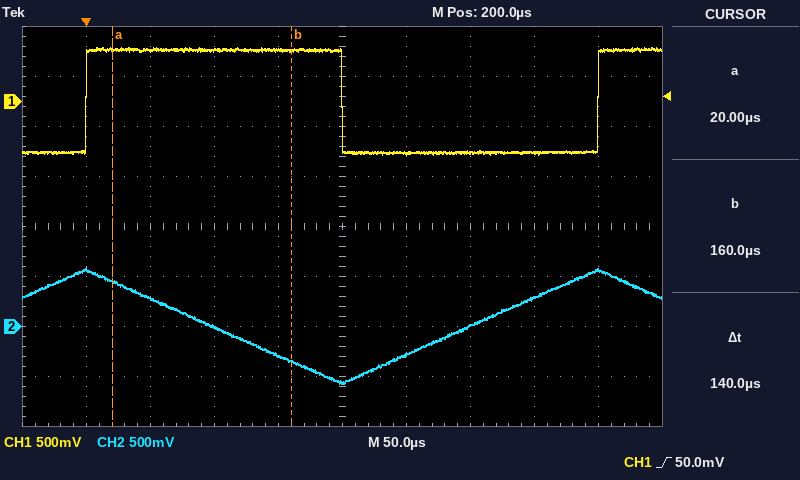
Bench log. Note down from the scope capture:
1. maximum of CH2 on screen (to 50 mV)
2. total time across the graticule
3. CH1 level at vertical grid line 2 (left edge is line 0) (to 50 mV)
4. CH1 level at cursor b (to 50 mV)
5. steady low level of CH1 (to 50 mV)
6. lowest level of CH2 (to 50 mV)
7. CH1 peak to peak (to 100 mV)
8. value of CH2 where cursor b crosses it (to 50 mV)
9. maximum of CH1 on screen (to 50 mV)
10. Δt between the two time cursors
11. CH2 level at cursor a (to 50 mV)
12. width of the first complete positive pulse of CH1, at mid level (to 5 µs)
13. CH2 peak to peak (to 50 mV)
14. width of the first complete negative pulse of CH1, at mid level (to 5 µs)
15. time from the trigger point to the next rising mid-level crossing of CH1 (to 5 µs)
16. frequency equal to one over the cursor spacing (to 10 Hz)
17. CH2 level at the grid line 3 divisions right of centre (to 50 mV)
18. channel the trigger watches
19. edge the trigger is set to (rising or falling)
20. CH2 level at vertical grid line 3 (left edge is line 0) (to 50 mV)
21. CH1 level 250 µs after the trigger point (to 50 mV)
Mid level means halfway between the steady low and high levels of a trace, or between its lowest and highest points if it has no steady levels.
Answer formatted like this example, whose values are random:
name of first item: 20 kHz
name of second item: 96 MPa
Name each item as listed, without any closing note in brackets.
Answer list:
maximum of CH2 on screen: 600 mV
total time across the graticule: 500 µs
CH1 level at vertical grid line 2 (left edge is line 0): 500 mV
CH1 level at cursor b: 500 mV
steady low level of CH1: -500 mV
lowest level of CH2: -550 mV
CH1 peak to peak: 1.10 V
value of CH2 where cursor b crosses it: -350 mV
maximum of CH1 on screen: 550 mV
Δt between the two time cursors: 140 µs
CH2 level at cursor a: 450 mV
width of the first complete positive pulse of CH1, at mid level: 200 µs
CH2 peak to peak: 1.15 V
width of the first complete negative pulse of CH1, at mid level: 200 µs
time from the trigger point to the next rising mid-level crossing of CH1: 400 µs
frequency equal to one over the cursor spacing: 7.14 kHz
CH2 level at the grid line 3 divisions right of centre: 300 mV
channel the trigger watches: CH1
edge the trigger is set to: rising
CH2 level at vertical grid line 3 (left edge is line 0): 0 mV
CH1 level 250 µs after the trigger point: -500 mV
